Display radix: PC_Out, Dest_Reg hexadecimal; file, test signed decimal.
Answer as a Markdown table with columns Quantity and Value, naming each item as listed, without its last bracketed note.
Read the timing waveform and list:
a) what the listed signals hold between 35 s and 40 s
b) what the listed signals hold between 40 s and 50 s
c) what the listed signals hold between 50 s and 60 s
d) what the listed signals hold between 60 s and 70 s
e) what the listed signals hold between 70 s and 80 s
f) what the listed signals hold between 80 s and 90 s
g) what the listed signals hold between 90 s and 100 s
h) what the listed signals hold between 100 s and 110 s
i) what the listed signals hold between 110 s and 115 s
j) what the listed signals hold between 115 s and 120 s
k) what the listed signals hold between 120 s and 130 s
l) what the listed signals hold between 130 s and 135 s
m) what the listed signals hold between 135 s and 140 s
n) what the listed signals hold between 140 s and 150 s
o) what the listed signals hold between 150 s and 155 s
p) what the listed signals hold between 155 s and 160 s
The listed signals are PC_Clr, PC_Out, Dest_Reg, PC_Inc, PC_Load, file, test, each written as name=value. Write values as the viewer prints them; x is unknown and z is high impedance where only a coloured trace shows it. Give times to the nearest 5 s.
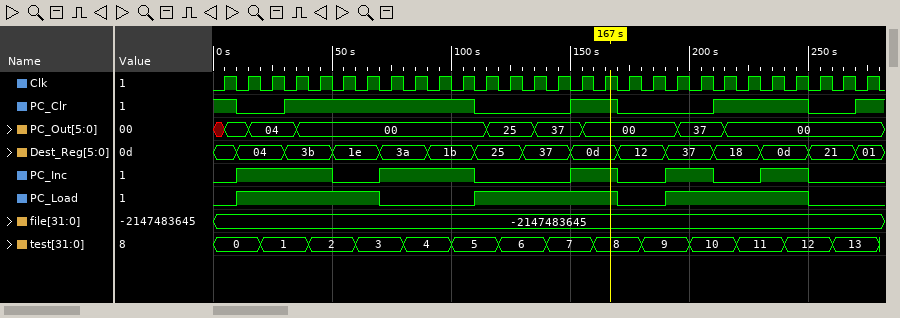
| Quantity | Value |
|---|---|
| what the listed signals hold between 35 s and 40 s | PC_Clr=1, PC_Out=00, Dest_Reg=3b, PC_Inc=1, PC_Load=1, file=-2147483645, test=1 |
| what the listed signals hold between 40 s and 50 s | PC_Clr=1, PC_Out=00, Dest_Reg=3b, PC_Inc=1, PC_Load=1, file=-2147483645, test=2 |
| what the listed signals hold between 50 s and 60 s | PC_Clr=1, PC_Out=00, Dest_Reg=1e, PC_Inc=0, PC_Load=1, file=-2147483645, test=2 |
| what the listed signals hold between 60 s and 70 s | PC_Clr=1, PC_Out=00, Dest_Reg=1e, PC_Inc=0, PC_Load=1, file=-2147483645, test=3 |
| what the listed signals hold between 70 s and 80 s | PC_Clr=1, PC_Out=00, Dest_Reg=3a, PC_Inc=1, PC_Load=0, file=-2147483645, test=3 |
| what the listed signals hold between 80 s and 90 s | PC_Clr=1, PC_Out=00, Dest_Reg=3a, PC_Inc=1, PC_Load=0, file=-2147483645, test=4 |
| what the listed signals hold between 90 s and 100 s | PC_Clr=1, PC_Out=00, Dest_Reg=1b, PC_Inc=1, PC_Load=0, file=-2147483645, test=4 |
| what the listed signals hold between 100 s and 110 s | PC_Clr=1, PC_Out=00, Dest_Reg=1b, PC_Inc=1, PC_Load=0, file=-2147483645, test=5 |
| what the listed signals hold between 110 s and 115 s | PC_Clr=0, PC_Out=00, Dest_Reg=25, PC_Inc=0, PC_Load=1, file=-2147483645, test=5 |
| what the listed signals hold between 115 s and 120 s | PC_Clr=0, PC_Out=25, Dest_Reg=25, PC_Inc=0, PC_Load=1, file=-2147483645, test=5 |
| what the listed signals hold between 120 s and 130 s | PC_Clr=0, PC_Out=25, Dest_Reg=25, PC_Inc=0, PC_Load=1, file=-2147483645, test=6 |
| what the listed signals hold between 130 s and 135 s | PC_Clr=0, PC_Out=25, Dest_Reg=37, PC_Inc=0, PC_Load=1, file=-2147483645, test=6 |
| what the listed signals hold between 135 s and 140 s | PC_Clr=0, PC_Out=37, Dest_Reg=37, PC_Inc=0, PC_Load=1, file=-2147483645, test=6 |
| what the listed signals hold between 140 s and 150 s | PC_Clr=0, PC_Out=37, Dest_Reg=37, PC_Inc=0, PC_Load=1, file=-2147483645, test=7 |
| what the listed signals hold between 150 s and 155 s | PC_Clr=1, PC_Out=37, Dest_Reg=0d, PC_Inc=1, PC_Load=1, file=-2147483645, test=7 |
| what the listed signals hold between 155 s and 160 s | PC_Clr=1, PC_Out=00, Dest_Reg=0d, PC_Inc=1, PC_Load=1, file=-2147483645, test=7 |
